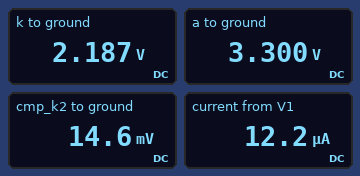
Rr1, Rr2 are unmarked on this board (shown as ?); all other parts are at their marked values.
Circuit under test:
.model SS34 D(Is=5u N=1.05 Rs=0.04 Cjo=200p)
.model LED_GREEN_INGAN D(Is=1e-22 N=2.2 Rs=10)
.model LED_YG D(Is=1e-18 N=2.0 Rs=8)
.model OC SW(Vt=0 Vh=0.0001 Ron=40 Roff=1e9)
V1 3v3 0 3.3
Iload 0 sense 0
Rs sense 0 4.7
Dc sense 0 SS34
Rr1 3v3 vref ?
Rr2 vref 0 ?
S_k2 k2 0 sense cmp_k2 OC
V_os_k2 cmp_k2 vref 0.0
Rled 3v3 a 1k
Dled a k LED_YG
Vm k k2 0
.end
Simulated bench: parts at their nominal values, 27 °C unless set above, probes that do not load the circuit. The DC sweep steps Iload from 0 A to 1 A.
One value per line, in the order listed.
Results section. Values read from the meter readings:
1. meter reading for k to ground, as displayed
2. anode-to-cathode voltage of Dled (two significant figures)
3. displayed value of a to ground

2.187 V
1.1 V
3.300 V
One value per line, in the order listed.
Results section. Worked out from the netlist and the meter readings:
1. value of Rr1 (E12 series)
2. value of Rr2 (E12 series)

270 kΩ
1.2 kΩ
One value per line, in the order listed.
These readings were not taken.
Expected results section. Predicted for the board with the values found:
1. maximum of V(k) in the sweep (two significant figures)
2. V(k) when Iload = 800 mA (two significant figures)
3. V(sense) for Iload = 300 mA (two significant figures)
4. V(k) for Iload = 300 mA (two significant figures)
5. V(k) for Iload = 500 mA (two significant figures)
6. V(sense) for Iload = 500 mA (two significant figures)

2.2 V
57 mV
300 mV
57 mV
57 mV
330 mV
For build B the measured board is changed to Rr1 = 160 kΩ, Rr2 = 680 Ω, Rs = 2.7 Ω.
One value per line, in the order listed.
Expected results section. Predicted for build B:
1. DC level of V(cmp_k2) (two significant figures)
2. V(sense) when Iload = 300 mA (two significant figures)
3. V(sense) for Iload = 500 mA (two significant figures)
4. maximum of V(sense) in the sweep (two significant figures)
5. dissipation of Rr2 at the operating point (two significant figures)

14 mV
290 mV
320 mV
360 mV
290 nW
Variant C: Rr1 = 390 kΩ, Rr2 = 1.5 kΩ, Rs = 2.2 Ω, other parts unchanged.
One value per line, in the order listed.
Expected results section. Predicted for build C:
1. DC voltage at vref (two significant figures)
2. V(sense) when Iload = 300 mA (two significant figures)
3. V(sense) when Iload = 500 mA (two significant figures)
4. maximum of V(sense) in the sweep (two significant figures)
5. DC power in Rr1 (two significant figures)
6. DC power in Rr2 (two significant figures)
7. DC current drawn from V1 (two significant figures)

13 mV
290 mV
320 mV
360 mV
28 µW
110 nW
8.4 µA
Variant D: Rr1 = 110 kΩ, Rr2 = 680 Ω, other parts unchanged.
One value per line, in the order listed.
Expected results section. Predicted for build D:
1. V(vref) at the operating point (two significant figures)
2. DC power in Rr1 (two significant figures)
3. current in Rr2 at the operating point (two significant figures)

20 mV
98 µW
30 µA
